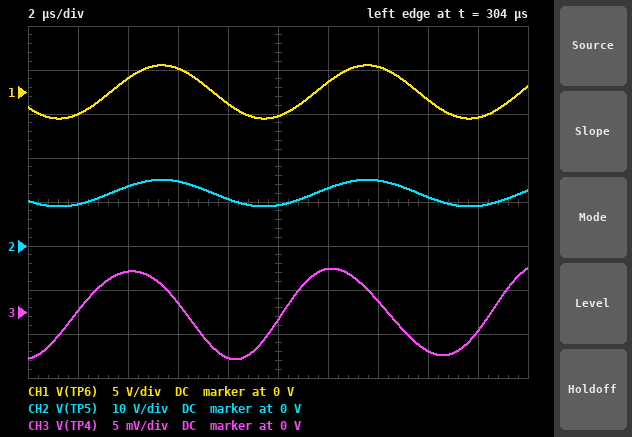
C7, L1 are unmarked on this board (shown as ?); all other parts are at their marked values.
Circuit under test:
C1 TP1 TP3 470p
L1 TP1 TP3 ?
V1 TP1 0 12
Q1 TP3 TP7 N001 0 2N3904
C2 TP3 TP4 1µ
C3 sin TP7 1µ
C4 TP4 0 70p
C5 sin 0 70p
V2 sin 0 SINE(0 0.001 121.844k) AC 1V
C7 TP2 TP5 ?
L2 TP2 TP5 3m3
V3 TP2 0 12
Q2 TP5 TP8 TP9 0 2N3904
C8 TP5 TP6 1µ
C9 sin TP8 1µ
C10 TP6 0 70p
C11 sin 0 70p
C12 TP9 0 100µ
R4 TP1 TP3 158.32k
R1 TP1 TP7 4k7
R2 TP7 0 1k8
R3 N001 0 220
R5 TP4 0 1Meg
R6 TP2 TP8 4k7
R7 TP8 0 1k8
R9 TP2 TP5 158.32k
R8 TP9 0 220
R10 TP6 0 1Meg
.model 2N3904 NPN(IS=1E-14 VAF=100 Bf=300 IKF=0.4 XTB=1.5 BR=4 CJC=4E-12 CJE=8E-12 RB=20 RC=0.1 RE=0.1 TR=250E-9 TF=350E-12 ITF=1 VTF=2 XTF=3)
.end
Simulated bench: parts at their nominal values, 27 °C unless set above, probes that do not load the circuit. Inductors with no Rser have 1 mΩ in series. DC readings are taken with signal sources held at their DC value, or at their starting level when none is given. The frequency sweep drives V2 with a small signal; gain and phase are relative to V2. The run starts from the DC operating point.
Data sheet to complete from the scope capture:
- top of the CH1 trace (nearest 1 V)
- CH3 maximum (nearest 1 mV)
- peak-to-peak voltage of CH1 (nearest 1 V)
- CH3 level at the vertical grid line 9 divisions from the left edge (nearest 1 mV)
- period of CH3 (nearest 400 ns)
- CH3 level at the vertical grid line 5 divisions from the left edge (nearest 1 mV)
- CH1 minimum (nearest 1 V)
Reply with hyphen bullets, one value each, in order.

- 3 V
- 5 mV
- 6 V
- -2 mV
- 8.4 µs
- -1 mV
- -3 V
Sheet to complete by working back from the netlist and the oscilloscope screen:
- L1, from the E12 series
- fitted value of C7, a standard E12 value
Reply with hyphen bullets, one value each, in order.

- 1 mH
- 330 pF
